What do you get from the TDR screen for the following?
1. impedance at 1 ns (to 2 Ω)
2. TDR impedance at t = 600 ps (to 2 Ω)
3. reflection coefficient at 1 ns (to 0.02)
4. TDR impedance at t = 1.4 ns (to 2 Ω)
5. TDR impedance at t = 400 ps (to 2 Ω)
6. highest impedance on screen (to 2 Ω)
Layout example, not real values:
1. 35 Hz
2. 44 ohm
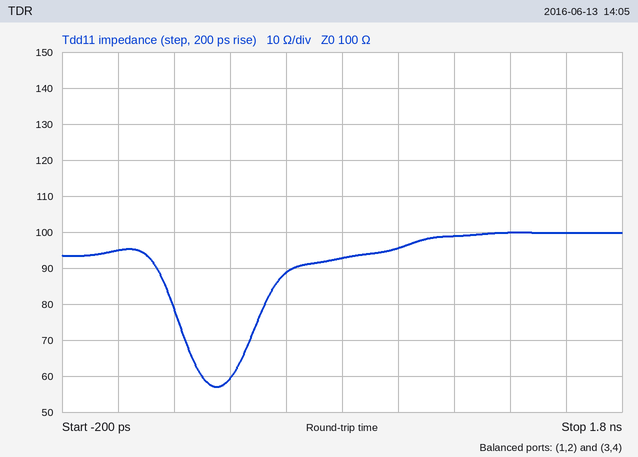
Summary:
1. 96 Ω
2. 88 Ω
3. -0.02
4. 100 Ω
5. 60 Ω
6. 100 Ω
